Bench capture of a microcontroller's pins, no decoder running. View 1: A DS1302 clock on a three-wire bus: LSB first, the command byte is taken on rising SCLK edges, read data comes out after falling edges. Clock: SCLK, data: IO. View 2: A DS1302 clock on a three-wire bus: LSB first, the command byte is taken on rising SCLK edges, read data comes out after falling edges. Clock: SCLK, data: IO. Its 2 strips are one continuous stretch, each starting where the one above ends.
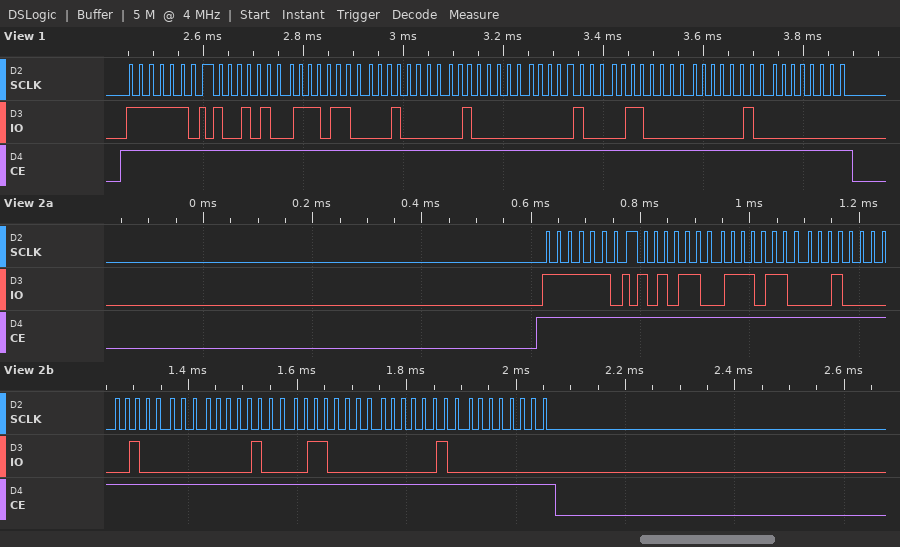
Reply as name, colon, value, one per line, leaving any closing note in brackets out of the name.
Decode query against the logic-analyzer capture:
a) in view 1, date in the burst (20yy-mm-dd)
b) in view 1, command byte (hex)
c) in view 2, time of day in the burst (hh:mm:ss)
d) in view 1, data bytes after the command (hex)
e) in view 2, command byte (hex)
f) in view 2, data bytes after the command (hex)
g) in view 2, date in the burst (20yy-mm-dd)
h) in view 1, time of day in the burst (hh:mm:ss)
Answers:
in view 1, date in the burst: 2020-10-02
in view 1, command byte: 0xBF
in view 2, time of day in the burst: 04:37:35
in view 1, data bytes after the command: 29 37 04 02 10 06 20 00
in view 2, command byte: 0xBF
in view 2, data bytes after the command: 35 37 04 02 10 06 20 00
in view 2, date in the burst: 2020-10-02
in view 1, time of day in the burst: 04:37:29
